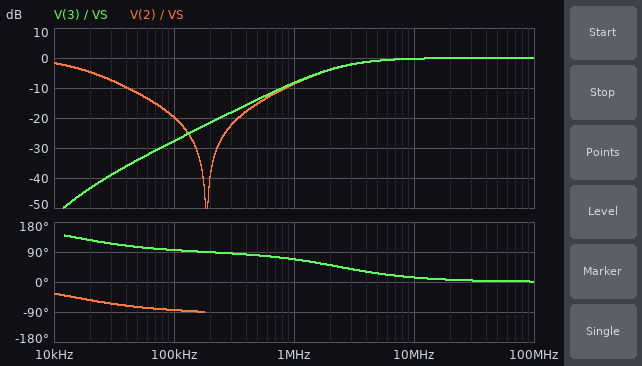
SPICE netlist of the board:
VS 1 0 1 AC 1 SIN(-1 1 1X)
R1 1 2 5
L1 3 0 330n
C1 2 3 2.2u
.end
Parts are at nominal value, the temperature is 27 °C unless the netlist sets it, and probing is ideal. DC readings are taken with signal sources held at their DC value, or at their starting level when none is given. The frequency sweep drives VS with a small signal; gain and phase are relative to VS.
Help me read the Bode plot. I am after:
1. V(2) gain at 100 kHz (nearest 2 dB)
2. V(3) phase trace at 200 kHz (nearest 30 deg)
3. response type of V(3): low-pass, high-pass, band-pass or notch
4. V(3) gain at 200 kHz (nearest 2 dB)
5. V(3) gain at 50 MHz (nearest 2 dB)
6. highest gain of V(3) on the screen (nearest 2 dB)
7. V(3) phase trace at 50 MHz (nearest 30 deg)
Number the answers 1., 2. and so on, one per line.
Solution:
1. -20 dB
2. 90 deg
3. high-pass
4. -22 dB
5. 0 dB
6. 0 dB
7. 0 deg
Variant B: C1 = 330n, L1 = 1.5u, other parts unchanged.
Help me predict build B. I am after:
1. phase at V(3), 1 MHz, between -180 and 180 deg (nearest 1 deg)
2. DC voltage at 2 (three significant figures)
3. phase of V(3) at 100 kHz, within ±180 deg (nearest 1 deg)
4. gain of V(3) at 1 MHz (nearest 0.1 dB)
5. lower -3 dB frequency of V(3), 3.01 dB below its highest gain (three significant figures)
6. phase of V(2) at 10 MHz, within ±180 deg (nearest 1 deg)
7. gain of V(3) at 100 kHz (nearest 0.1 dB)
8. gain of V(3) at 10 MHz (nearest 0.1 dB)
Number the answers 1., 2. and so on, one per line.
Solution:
1. 29 deg
2. 1.00 V
3. 128 deg
4. -0.7 dB
5. 439 kHz
6. 3 deg
7. -16.5 dB
8. 0 dB
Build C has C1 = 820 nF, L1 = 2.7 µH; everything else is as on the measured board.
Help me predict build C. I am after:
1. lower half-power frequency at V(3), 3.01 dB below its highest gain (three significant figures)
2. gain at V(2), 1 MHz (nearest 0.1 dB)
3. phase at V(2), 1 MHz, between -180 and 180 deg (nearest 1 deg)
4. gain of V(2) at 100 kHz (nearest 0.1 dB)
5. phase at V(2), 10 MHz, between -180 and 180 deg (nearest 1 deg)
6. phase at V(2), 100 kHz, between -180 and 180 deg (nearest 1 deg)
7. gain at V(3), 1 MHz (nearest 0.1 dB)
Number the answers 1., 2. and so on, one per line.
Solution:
1. 257 kHz
2. -0.4 dB
3. 17 deg
4. -26.2 dB
5. 2 deg
6. -87 deg
7. -0.3 dB
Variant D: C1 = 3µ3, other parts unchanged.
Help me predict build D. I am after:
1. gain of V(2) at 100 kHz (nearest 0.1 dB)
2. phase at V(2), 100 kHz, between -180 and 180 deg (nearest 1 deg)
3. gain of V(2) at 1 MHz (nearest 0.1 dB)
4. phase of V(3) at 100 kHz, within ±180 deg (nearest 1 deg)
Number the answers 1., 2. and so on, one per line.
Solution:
1. -25.2 dB
2. -87 deg
3. -8.5 dB
4. 93 deg
